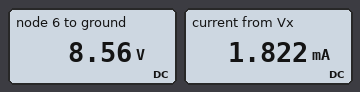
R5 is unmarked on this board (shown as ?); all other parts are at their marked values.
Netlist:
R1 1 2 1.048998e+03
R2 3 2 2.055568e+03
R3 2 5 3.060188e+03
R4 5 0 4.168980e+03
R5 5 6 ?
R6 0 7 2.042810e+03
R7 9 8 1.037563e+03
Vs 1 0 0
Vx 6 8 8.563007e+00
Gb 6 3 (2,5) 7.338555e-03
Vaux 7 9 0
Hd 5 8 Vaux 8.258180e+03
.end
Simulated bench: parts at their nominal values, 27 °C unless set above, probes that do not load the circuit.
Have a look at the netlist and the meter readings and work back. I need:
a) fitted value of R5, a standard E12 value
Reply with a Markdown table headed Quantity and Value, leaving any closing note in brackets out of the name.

| Quantity | Value |
|---|---|
| fitted value of R5, a standard E12 value | 4.7 kΩ |
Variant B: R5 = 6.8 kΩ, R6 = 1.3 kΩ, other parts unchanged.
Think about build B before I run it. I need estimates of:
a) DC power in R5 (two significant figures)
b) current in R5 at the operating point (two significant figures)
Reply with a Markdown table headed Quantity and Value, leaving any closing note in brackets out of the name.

| Quantity | Value |
|---|---|
| DC power in R5 | 11 mW |
| current in R5 at the operating point | 1.3 mA |
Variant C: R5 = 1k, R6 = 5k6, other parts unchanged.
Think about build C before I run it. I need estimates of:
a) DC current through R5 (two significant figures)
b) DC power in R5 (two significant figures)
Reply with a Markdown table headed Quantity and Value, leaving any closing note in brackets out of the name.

| Quantity | Value |
|---|---|
| DC current through R5 | 8.6 mA |
| DC power in R5 | 73 mW |
